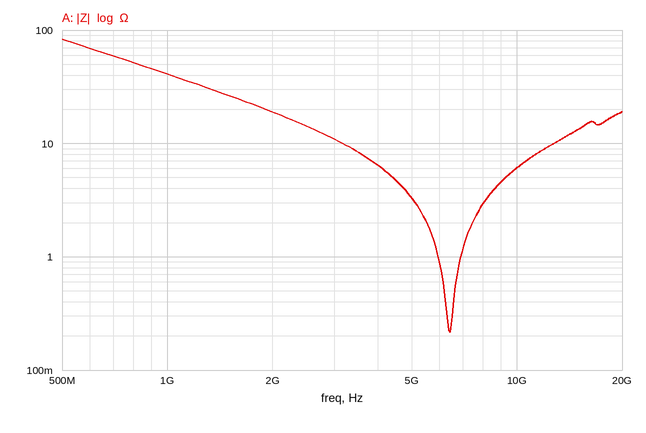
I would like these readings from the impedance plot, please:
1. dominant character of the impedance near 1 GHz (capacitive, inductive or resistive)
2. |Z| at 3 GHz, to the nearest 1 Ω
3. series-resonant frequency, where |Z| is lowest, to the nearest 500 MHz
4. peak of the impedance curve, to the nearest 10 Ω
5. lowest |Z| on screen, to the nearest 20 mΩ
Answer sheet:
capacitive
11 Ω
6.5 GHz
80 Ω
220 mΩ
